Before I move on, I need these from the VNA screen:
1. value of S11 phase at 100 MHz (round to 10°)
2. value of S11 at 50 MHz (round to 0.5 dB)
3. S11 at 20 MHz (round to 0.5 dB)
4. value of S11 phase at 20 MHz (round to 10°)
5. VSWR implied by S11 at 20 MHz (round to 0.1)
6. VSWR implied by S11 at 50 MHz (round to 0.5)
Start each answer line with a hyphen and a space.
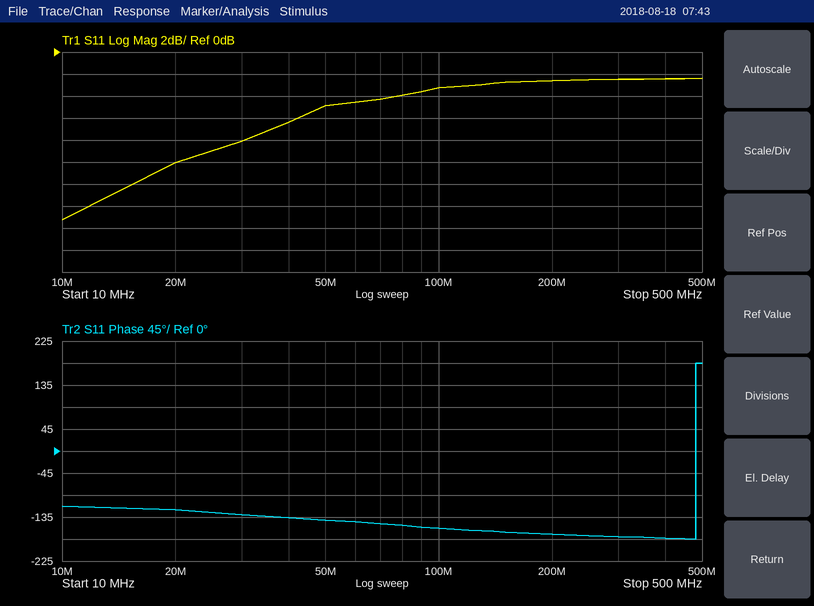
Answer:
- -160°
- -5.0 dB
- -10.0 dB
- -120°
- 1.9
- 3.5
